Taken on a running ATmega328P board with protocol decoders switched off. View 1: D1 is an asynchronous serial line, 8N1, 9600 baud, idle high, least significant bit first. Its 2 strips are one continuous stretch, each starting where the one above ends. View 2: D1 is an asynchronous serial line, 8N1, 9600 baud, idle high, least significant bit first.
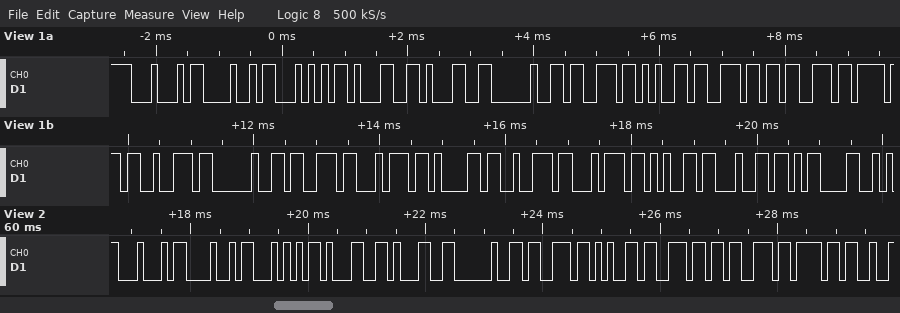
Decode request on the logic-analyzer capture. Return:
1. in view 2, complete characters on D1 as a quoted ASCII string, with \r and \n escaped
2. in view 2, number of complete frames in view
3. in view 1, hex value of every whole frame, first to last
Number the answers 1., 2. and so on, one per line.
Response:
1. "DHT11 senso"
2. 11
3. 44 48 54 31 31 20 73 65 6E 73 6F 72 20 73 74 61 72 74 65 64 0D
